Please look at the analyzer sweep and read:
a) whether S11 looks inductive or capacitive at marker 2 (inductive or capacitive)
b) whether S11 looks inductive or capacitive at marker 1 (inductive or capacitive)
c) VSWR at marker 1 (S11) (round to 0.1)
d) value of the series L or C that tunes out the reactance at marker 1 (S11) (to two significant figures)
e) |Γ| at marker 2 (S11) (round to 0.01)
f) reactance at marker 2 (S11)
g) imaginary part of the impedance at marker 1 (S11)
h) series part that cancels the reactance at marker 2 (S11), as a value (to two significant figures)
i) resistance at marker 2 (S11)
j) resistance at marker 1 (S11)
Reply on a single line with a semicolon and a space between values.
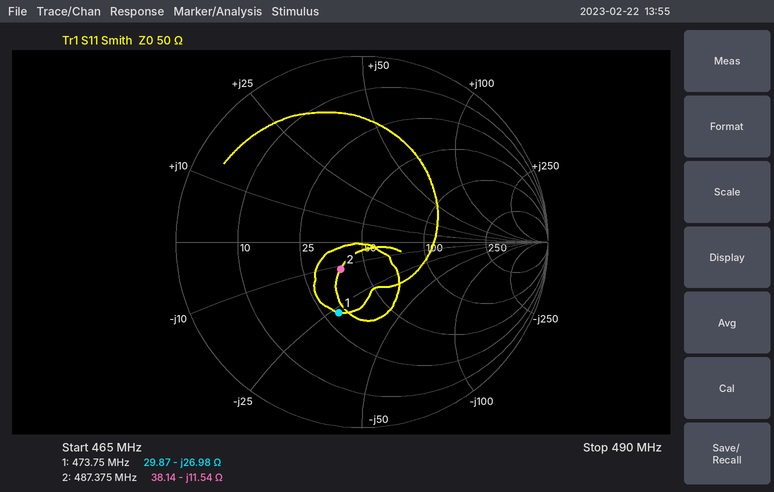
capacitive; capacitive; 2.3; 9.1 nH; 0.19; -11.54 Ω; -26.98 Ω; 3.8 nH; 38.14 Ω; 29.87 Ω
